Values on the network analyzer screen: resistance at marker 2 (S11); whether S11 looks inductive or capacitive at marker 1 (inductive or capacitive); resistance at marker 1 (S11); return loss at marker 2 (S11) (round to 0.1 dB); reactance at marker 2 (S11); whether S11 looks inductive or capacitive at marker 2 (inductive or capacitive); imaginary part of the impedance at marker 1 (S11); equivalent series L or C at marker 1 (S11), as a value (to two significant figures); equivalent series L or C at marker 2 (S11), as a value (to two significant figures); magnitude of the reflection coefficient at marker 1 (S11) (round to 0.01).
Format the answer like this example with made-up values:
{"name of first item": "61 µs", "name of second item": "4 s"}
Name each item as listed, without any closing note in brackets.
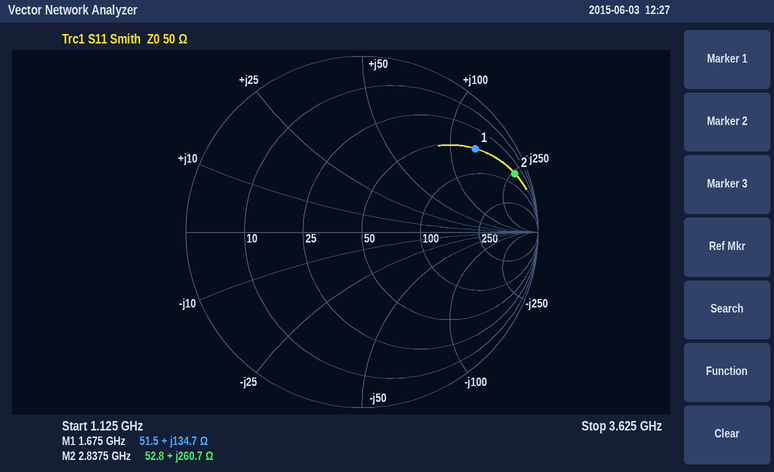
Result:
{"resistance at marker 2": "52.8 Ω", "whether S11 looks inductive or capacitive at marker 1": "inductive", "resistance at marker 1": "51.5 Ω", "return loss at marker 2 (S11)": "0.6 dB", "reactance at marker 2": "+260.7 Ω", "whether S11 looks inductive or capacitive at marker 2": "inductive", "imaginary part of the impedance at marker 1": "+134.7 Ω", "equivalent series L or C at marker 1 (S11), as a value": "13 nH", "equivalent series L or C at marker 2 (S11), as a value": "15 nH", "magnitude of the reflection coefficient at marker 1 (S11)": "0.80"}
